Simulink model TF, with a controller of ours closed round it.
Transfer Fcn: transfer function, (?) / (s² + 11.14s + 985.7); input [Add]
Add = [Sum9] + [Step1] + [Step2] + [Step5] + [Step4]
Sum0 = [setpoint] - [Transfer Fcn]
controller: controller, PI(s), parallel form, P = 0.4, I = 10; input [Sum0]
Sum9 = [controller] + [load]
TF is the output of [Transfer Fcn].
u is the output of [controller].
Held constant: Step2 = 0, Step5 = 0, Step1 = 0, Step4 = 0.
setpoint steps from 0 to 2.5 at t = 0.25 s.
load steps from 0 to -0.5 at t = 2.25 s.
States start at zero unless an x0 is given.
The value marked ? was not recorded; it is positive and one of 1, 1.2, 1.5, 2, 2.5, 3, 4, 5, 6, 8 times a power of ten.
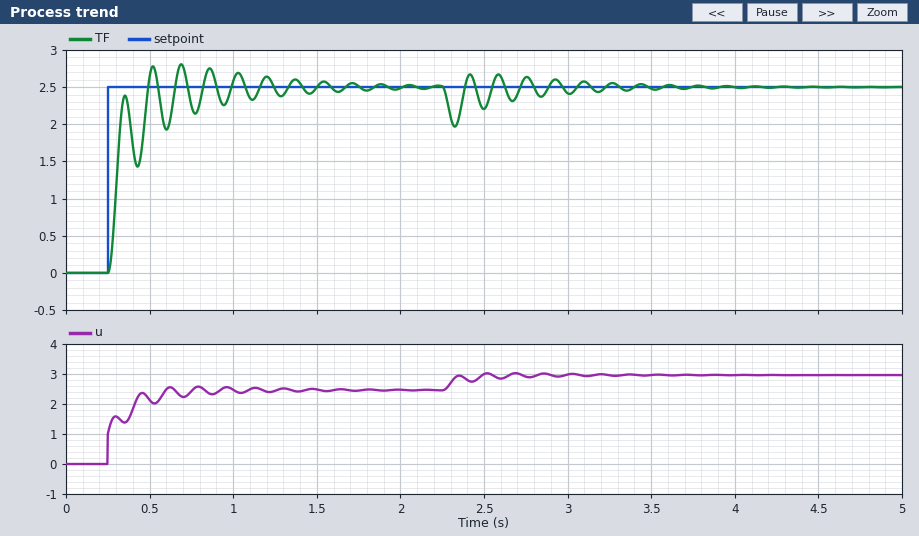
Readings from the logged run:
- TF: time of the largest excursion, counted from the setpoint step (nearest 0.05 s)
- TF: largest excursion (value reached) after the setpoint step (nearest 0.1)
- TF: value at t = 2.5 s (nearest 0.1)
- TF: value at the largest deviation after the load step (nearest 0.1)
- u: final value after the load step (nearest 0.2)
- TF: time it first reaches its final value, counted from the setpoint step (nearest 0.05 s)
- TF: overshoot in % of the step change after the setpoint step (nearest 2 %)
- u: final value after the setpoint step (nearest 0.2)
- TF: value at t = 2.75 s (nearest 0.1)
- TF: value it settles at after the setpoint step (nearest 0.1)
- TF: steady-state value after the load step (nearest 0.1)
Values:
0.45 s
2.8
2.2
2.0
3.0
0.25 s
12 %
2.4
2.6
2.5
2.5
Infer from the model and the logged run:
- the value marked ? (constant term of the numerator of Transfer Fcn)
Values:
1000
